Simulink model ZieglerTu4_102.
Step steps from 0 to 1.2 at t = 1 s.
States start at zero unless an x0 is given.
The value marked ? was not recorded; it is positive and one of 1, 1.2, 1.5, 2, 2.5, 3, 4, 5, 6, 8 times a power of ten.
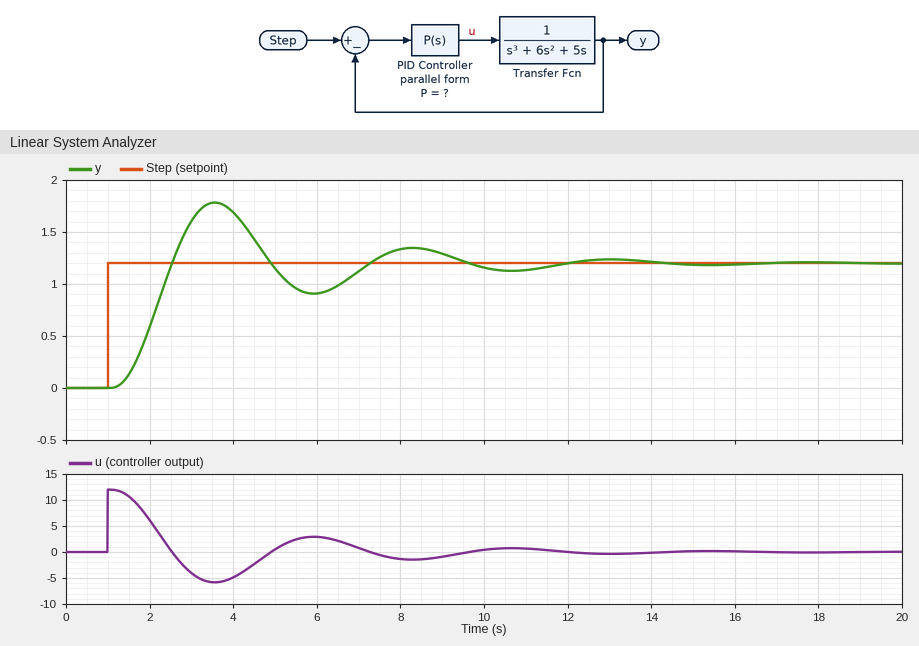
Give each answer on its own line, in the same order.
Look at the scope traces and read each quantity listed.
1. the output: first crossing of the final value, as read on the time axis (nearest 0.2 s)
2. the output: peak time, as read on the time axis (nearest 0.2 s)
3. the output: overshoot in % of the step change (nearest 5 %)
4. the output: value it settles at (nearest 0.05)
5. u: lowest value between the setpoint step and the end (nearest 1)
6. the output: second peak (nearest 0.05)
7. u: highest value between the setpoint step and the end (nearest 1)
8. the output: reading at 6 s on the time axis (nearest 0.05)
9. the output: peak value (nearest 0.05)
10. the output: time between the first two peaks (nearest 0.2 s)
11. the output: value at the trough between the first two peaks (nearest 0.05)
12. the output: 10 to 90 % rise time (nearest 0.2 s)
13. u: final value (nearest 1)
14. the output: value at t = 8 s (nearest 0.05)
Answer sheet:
2.6 s
3.6 s
50 %
1.20
-6
1.35
12
0.90
1.80
4.8 s
0.90
1.0 s
0
1.35
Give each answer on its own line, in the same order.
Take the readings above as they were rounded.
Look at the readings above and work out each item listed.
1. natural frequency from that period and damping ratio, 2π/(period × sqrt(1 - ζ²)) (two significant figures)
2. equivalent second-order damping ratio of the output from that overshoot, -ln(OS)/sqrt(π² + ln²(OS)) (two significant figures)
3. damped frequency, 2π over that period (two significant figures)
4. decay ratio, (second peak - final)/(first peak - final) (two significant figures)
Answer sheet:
1.3 rad/s
0.22
1.3 rad/s
0.25
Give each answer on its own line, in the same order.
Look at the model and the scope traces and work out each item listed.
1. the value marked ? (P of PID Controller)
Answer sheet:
10
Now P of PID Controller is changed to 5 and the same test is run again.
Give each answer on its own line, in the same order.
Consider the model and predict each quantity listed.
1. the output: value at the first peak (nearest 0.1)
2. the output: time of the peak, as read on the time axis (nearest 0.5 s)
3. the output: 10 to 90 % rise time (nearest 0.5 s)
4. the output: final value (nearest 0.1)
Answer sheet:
1.5
4.5 s
1.5 s
1.2
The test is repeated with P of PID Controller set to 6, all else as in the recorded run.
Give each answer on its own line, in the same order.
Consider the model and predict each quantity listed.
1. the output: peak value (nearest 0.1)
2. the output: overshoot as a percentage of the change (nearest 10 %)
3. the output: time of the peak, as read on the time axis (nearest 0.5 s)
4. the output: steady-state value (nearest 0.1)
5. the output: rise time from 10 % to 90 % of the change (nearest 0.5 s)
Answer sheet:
1.6
30 %
4.5 s
1.2
1.5 s
